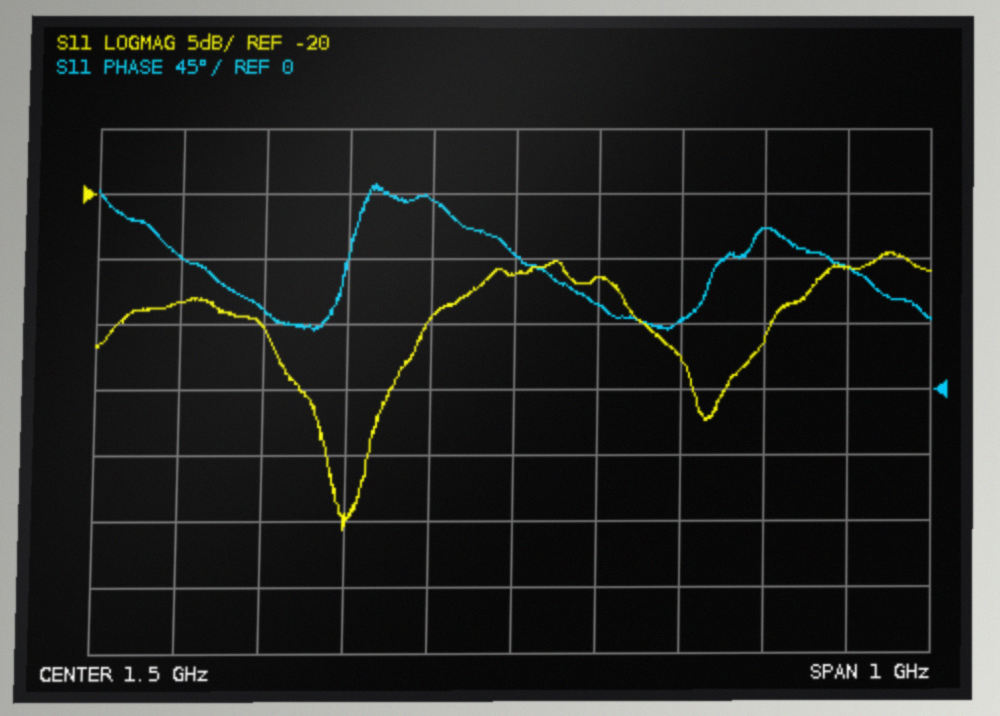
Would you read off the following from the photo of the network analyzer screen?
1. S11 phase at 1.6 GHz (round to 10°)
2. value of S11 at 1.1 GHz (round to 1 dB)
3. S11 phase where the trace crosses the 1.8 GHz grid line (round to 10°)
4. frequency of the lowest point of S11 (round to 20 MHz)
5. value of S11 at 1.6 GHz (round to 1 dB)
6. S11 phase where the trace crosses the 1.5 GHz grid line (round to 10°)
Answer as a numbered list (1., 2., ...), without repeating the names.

1. 60°
2. -28 dB
3. 110°
4. 1.30 GHz
5. -26 dB
6. 90°
